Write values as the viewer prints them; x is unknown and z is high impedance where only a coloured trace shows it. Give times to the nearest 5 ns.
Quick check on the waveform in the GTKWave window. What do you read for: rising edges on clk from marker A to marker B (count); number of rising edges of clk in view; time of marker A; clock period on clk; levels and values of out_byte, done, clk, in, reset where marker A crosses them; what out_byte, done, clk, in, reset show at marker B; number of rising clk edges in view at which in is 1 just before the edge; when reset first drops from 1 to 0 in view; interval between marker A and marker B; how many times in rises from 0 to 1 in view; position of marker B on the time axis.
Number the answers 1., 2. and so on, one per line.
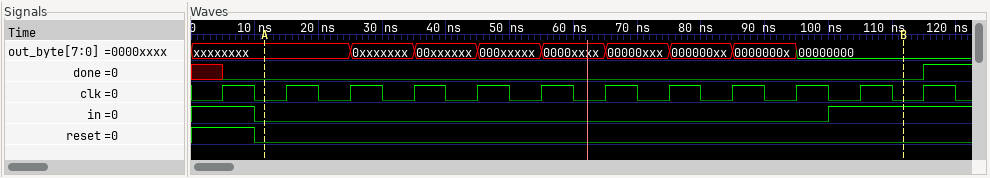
1. 10
2. 12
3. 10 ns
4. 10 ns
5. out_byte=xxxxxxxx, done=0, clk=0, in=0, reset=0
6. out_byte=00000000, done=0, clk=0, in=1, reset=0
7. 3
8. 10 ns
9. 100 ns
10. 1
11. 110 ns
